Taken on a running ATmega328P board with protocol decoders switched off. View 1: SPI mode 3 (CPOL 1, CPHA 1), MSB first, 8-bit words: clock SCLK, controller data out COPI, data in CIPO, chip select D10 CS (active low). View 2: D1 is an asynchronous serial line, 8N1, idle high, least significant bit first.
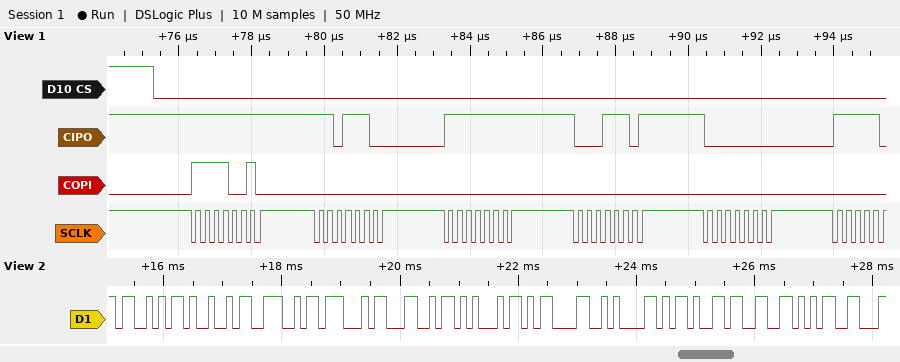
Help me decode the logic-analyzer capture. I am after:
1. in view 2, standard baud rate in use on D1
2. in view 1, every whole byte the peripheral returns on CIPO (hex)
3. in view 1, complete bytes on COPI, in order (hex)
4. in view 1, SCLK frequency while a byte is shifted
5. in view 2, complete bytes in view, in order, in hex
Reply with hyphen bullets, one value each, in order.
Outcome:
- 9600 baud
- FF DC FF 1D 00
- F2 00 00 00 00
- 4 MHz
- 53 49 4E 47 4C 45 0D 0A 2D 33 35
